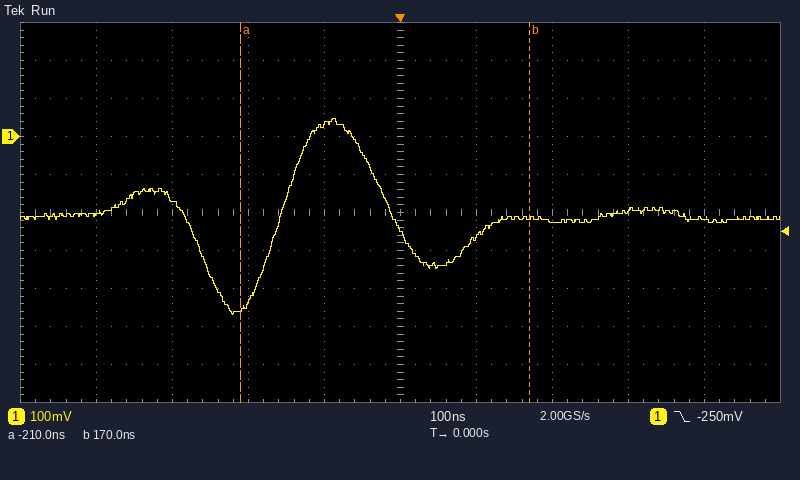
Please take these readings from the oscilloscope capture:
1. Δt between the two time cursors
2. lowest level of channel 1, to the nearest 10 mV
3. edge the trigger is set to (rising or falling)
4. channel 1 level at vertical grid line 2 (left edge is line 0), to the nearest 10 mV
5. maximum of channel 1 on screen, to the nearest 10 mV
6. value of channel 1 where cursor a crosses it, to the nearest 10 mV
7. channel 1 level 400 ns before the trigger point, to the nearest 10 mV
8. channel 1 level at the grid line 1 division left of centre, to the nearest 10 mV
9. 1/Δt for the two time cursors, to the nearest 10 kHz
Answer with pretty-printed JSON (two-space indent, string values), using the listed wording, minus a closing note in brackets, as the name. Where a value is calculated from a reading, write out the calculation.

{
  "Δt between the two time cursors": "170 ns − (-210 ns) = 380 ns",
  "lowest level of channel 1, to the nearest 10 mV": "-470 mV",
  "edge the trigger is set to": "falling",
  "channel 1 level at vertical grid line 2 (left edge is line 0), to the nearest 10 mV": "-160 mV",
  "maximum of channel 1 on screen, to the nearest 10 mV": "50 mV",
  "value of channel 1 where cursor a crosses it, to the nearest 10 mV": "-450 mV",
  "channel 1 level 400 ns before the trigger point, to the nearest 10 mV": "-200 mV",
  "channel 1 level at the grid line 1 division left of centre, to the nearest 10 mV": "30 mV",
  "1/Δt for the two time cursors, to the nearest 10 kHz": "1 / 380 ns ≈ 2.63 MHz"
}
